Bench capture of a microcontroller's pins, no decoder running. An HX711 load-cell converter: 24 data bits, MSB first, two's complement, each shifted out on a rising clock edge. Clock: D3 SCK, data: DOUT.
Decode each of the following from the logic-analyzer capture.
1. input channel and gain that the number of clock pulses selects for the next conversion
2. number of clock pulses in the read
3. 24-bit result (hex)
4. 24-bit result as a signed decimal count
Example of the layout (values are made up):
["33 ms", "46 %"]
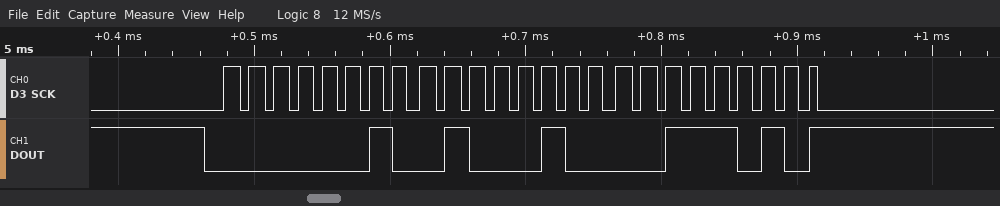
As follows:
["channel A, gain 128", "25", "0x02443A", "148538"]
